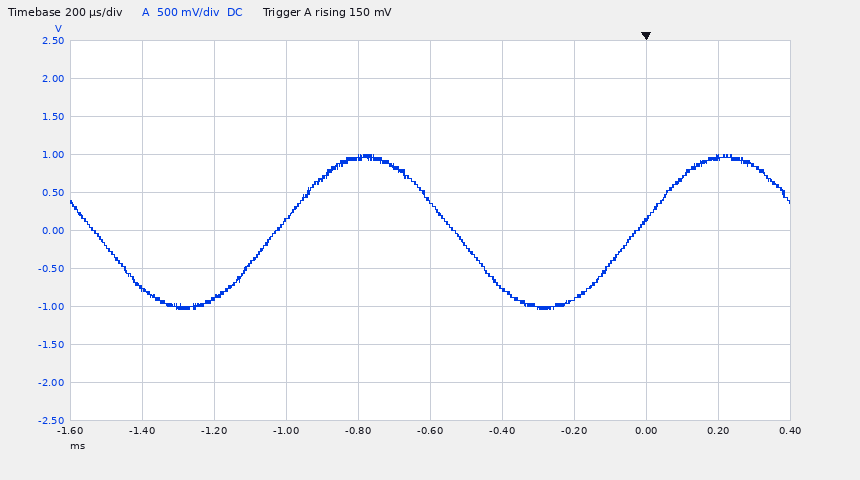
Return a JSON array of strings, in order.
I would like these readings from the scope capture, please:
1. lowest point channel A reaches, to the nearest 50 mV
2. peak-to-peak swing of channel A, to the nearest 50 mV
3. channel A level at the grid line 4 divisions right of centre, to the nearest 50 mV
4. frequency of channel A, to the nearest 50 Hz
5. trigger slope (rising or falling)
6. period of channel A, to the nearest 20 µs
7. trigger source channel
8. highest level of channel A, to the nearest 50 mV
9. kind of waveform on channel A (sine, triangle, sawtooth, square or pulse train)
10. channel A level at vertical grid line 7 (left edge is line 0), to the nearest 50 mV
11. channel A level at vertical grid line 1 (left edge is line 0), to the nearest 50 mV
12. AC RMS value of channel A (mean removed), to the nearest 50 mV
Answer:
["-1.05 V", "2.05 V", "950 mV", "1.00 kHz", "rising", "1.00 ms", "channel A", "1.00 V", "sine", "-900 mV", "-750 mV", "700 mV"]
